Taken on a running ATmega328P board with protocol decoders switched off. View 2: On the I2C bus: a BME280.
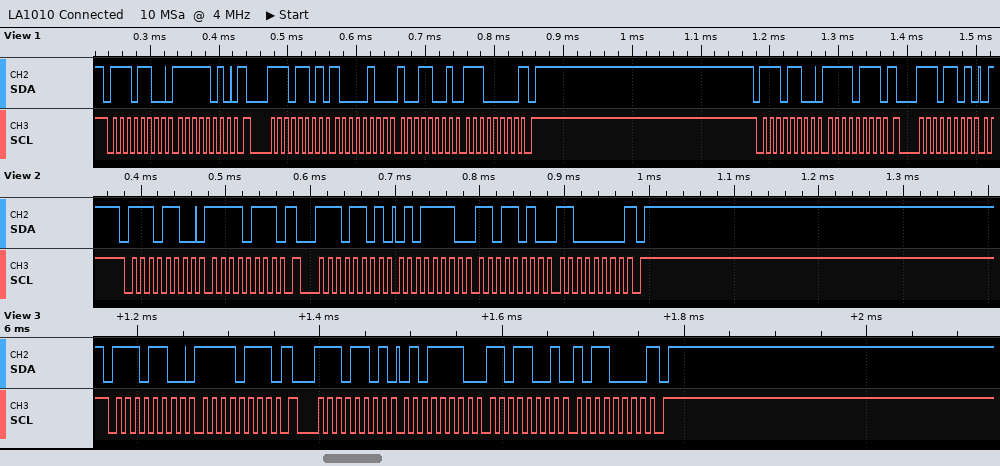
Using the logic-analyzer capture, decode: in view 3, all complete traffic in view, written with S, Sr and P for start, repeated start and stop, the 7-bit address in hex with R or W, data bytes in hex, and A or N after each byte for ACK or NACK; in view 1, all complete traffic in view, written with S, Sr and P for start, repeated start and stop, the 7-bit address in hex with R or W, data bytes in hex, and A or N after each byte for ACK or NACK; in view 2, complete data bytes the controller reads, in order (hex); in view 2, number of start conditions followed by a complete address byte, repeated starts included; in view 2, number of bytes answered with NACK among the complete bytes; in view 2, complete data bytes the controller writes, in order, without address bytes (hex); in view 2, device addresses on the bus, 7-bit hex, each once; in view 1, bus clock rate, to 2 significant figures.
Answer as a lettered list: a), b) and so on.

a) S 76W A F7 A Sr 76R A 5E A D9 A B0 N P
b) S 76W A FA A Sr 76R A 84 A 99 A E0 N P S 76W A F7 A Sr 76R A
c) 5E DA C0
d) 2
e) 1
f) F7
g) 0x76
h) 100 kHz
